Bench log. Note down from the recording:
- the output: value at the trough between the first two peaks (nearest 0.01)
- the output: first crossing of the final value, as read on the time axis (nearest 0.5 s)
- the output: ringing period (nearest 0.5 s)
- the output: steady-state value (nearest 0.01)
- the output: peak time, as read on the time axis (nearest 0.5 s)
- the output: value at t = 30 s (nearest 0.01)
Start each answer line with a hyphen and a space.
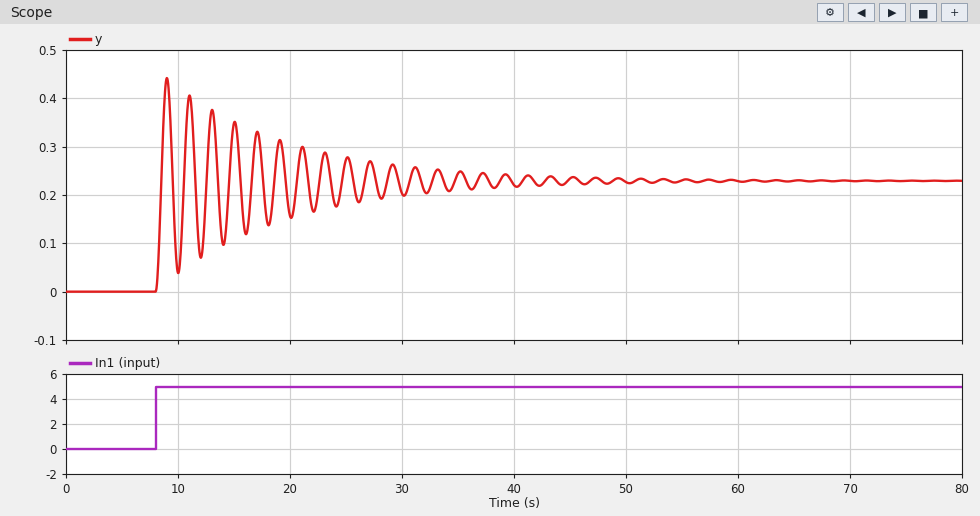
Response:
- 0.04
- 8.5 s
- 2.0 s
- 0.23
- 9.0 s
- 0.20
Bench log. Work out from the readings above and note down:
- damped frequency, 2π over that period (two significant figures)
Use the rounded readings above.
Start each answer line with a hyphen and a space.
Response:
- 3.1 rad/s
